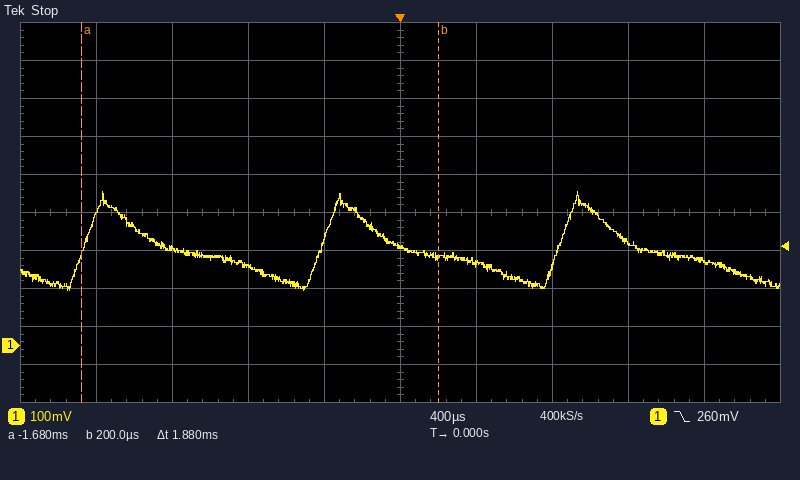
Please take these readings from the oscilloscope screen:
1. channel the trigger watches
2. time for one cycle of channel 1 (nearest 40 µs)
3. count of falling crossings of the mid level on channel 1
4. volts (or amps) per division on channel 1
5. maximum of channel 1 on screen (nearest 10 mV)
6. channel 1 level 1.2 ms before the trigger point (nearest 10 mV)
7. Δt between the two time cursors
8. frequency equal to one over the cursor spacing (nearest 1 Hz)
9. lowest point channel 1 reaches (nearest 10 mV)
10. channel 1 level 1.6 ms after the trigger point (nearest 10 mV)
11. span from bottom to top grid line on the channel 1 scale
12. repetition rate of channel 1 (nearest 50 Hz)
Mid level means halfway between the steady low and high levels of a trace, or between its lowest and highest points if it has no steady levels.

channel 1
1.24 ms
3
100 mV
410 mV
250 mV
1.88 ms
532 Hz
140 mV
220 mV
1 V
800 Hz
